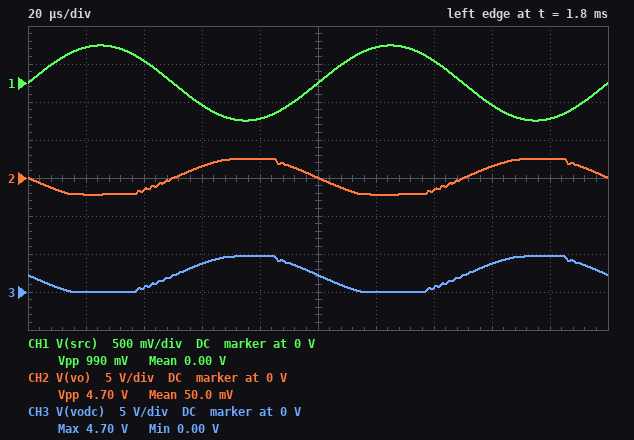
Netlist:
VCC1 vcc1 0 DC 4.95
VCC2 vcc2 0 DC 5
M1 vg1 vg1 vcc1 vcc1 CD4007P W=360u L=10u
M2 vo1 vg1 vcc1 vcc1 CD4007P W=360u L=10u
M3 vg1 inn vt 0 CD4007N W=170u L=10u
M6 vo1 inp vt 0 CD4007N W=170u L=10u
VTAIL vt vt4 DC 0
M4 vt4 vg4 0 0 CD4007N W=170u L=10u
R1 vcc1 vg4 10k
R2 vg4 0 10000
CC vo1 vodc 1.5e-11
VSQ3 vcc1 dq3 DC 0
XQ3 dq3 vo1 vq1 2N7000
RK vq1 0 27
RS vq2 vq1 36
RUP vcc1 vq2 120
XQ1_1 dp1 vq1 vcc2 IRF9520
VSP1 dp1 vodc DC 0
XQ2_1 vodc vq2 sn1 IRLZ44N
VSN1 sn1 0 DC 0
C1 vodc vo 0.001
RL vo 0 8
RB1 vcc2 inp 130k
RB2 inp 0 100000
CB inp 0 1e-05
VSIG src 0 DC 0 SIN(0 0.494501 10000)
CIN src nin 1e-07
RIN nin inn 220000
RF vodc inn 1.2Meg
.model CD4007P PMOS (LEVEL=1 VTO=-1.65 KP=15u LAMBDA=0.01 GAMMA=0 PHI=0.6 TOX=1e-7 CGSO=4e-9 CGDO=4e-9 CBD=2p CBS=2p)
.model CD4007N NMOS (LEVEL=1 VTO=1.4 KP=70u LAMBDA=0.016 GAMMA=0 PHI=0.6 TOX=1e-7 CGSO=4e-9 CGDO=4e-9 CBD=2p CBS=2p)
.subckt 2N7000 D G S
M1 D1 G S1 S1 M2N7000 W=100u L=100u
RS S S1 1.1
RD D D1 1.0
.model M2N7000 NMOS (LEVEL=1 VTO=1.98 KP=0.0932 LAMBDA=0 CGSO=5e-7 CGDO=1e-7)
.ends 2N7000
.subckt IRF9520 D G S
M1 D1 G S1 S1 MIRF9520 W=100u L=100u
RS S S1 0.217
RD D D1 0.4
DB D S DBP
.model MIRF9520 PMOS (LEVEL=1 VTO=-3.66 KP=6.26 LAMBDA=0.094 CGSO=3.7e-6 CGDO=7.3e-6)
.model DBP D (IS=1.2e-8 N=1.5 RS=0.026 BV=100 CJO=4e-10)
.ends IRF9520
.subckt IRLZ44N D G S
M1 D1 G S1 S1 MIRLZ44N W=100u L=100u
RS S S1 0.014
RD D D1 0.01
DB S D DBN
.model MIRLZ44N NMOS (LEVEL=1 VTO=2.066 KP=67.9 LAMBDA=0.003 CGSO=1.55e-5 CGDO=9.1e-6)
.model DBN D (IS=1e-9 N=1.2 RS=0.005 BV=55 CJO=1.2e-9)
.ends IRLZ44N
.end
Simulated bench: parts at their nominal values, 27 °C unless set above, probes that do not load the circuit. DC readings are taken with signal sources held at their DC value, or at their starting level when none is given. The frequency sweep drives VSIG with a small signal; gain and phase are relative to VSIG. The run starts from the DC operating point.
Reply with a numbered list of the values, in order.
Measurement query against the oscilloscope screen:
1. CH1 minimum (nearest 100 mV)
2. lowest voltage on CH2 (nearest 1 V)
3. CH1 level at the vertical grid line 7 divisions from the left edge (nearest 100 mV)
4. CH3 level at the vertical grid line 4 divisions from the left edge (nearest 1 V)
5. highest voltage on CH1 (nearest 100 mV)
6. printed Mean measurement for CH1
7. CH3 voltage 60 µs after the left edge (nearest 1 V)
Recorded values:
1. -500 mV
2. -2 V
3. 300 mV
4. 5 V
5. 500 mV
6. 0.00 V
7. 4 V
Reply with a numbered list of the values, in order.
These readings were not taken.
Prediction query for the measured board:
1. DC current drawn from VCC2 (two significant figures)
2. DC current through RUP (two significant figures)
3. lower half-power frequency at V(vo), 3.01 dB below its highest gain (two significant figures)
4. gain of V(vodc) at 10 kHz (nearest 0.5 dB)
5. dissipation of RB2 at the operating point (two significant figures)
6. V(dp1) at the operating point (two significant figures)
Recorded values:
1. 33 mA
2. 24 mA
3. 410 kHz
4. 14.5 dB
5. 47 µW
6. 2.2 V
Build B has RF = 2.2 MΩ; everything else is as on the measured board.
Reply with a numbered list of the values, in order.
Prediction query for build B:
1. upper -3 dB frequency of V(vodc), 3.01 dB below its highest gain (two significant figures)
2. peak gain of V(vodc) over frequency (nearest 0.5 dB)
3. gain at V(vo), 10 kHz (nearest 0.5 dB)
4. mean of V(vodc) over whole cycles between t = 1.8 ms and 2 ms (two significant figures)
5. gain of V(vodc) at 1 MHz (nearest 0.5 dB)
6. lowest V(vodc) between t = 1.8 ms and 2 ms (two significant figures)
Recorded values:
1. 400 kHz
2. 27.5 dB
3. 20.0 dB
4. 2.3 V
5. -0.5 dB
6. 17 mV
